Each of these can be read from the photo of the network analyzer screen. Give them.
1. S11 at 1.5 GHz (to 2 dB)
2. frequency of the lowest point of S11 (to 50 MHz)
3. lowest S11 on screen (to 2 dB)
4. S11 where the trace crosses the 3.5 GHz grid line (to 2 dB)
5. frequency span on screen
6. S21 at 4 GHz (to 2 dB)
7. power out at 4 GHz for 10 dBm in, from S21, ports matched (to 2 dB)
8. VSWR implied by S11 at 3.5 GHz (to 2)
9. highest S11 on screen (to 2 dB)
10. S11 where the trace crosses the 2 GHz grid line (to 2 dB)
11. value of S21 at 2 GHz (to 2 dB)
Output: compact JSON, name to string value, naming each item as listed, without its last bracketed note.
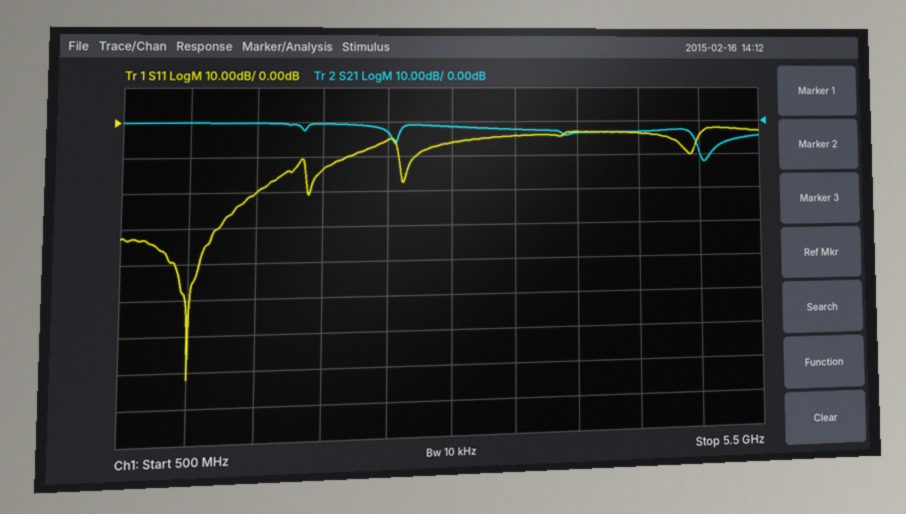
{"S11 at 1.5 GHz": "-20 dB", "frequency of the lowest point of S11": "1.00 GHz", "lowest S11 on screen": "-72 dB", "S11 where the trace crosses the 3.5 GHz grid line": "-4 dB", "frequency span on screen": "5 GHz", "S21 at 4 GHz": "-4 dB", "power out at 4 GHz for 10 dBm in, from S21, ports matched": "6 dBm", "VSWR implied by S11 at 3.5 GHz": "4", "highest S11 on screen": "-2 dB", "S11 where the trace crosses the 2 GHz grid line": "-14 dB", "value of S21 at 2 GHz": "0 dB"}
